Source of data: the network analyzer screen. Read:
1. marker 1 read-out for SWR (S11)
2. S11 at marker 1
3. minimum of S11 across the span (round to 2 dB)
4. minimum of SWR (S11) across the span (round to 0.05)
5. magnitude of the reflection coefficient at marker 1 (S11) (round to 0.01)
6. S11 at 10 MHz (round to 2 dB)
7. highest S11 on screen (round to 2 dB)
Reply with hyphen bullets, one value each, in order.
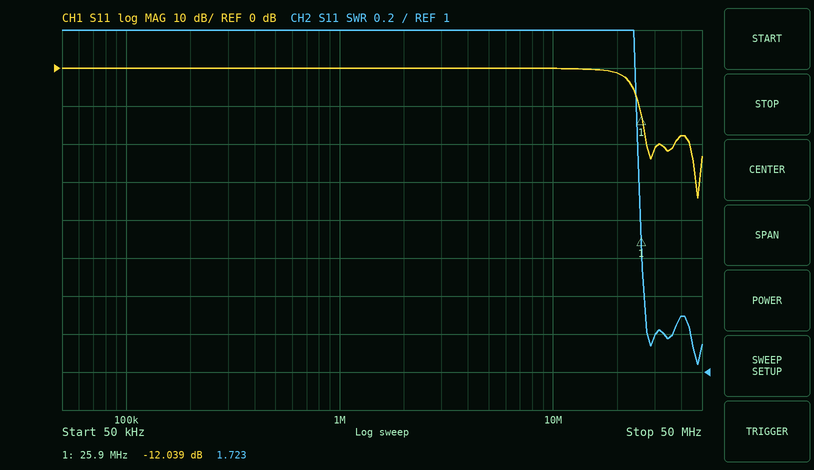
- 1.723
- -12.039 dB
- -34 dB
- 1.05
- 0.25
- 0 dB
- 0 dB
